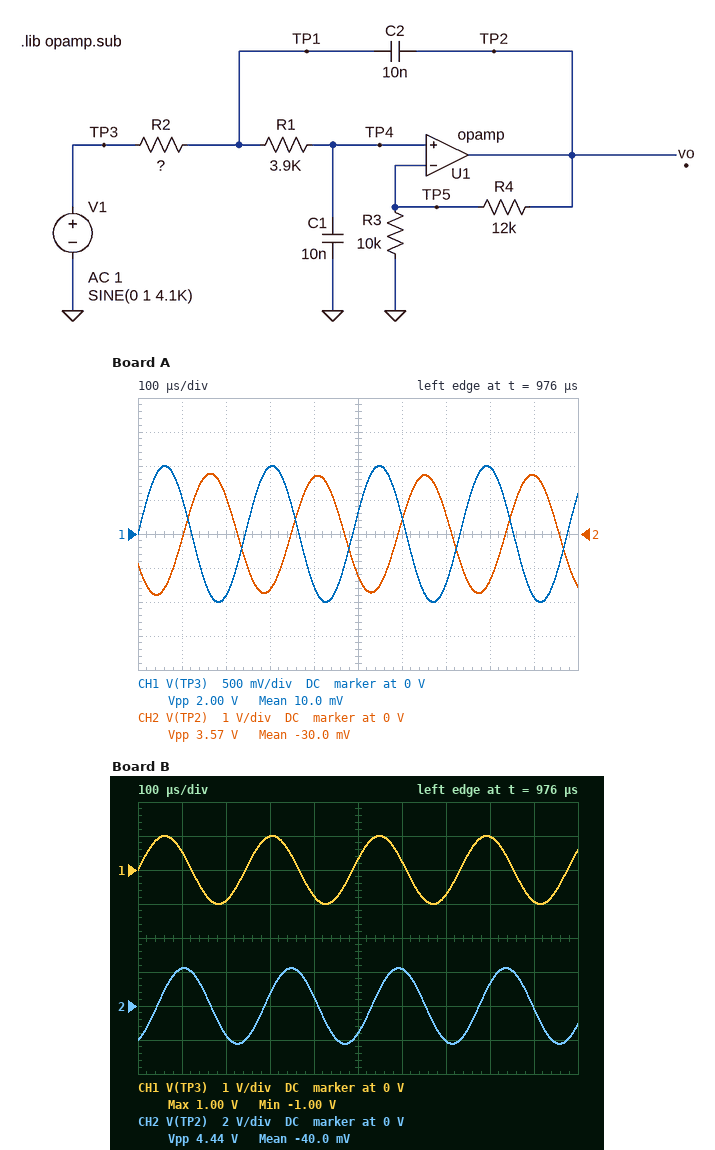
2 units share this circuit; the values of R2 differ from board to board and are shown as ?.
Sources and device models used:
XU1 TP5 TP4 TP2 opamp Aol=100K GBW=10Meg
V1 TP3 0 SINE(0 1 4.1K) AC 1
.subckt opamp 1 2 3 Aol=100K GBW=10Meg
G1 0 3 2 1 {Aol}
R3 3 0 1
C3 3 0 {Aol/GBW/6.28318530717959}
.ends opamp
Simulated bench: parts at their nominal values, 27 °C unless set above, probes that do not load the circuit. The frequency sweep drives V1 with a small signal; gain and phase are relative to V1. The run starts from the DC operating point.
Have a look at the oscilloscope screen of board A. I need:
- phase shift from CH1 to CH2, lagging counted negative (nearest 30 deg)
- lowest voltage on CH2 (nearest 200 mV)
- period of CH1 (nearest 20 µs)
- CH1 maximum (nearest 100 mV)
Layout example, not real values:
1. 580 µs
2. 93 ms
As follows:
1. -150 deg
2. -1.8 V
3. 240 µs
4. 1.0 V
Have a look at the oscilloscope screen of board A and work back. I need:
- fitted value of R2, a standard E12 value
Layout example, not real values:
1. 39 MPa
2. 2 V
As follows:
1. 8.2 kΩ
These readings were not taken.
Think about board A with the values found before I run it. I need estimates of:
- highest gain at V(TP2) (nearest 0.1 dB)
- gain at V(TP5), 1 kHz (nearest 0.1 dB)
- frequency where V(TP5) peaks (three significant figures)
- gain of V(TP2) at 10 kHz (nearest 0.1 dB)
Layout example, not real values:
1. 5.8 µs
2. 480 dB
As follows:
1. 15.0 dB
2. 1.1 dB
3. 2.70 kHz
4. -14.5 dB
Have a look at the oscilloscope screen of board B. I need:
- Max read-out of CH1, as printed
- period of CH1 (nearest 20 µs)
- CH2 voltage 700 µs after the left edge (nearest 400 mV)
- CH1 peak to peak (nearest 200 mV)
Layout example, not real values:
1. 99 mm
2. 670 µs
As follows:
1. 1.00 V
2. 240 µs
3. -2.0 V
4. 2.0 V
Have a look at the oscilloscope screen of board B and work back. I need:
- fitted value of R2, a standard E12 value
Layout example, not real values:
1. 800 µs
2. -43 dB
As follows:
1. 2.2 kΩ
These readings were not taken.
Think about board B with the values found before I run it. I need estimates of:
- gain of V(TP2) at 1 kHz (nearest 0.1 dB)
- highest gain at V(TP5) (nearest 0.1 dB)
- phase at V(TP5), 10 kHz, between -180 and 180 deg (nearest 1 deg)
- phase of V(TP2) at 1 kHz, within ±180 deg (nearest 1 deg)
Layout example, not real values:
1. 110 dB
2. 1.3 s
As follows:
1. 6.9 dB
2. 0.4 dB
3. -138 deg
4. -13 deg
